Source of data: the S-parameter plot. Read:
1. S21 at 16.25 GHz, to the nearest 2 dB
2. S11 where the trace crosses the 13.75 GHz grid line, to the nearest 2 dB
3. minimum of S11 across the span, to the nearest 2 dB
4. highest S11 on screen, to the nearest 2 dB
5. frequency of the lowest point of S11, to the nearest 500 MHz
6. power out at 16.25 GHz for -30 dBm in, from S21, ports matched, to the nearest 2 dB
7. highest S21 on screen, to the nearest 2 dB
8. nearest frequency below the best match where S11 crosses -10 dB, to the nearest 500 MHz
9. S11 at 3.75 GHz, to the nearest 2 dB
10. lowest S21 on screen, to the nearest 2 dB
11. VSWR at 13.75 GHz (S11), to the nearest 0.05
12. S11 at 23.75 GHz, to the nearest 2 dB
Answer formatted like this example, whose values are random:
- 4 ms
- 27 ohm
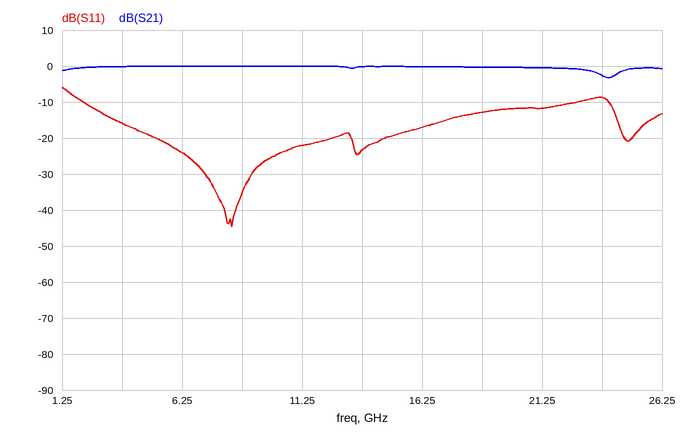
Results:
- 0 dB
- -24 dB
- -44 dB
- -6 dB
- 8.5 GHz
- -30 dBm
- 0 dB
- 2.0 GHz
- -16 dB
- -4 dB
- 1.15
- -8 dB
